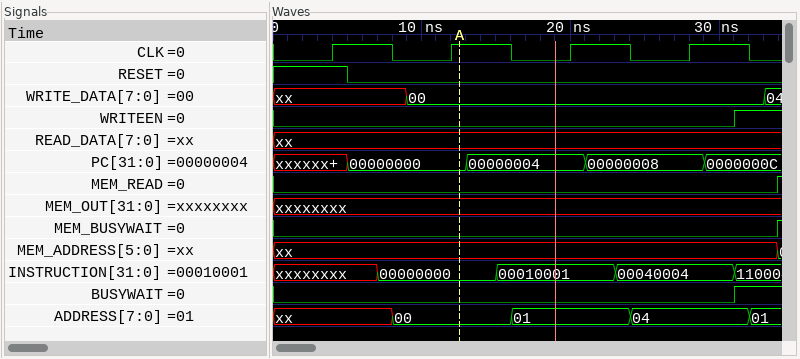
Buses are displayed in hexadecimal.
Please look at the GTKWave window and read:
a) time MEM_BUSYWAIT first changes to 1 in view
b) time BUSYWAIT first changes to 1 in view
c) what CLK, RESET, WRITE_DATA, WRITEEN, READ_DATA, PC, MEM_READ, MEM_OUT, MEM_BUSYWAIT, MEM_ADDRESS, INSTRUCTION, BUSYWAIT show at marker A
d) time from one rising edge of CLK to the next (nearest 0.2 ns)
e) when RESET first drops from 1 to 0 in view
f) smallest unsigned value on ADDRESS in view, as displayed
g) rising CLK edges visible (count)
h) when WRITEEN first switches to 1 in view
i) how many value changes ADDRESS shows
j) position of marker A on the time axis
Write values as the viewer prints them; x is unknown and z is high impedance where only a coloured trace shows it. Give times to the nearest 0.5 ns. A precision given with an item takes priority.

34 ns
31 ns
CLK=1, RESET=0, WRITE_DATA=00, WRITEEN=0, READ_DATA=xx, PC=00000000, MEM_READ=0, MEM_OUT=xxxxxxxx, MEM_BUSYWAIT=0, MEM_ADDRESS=xx, INSTRUCTION=00000000, BUSYWAIT=0
8 ns
5 ns
00
4
31 ns
4
12.5 ns
